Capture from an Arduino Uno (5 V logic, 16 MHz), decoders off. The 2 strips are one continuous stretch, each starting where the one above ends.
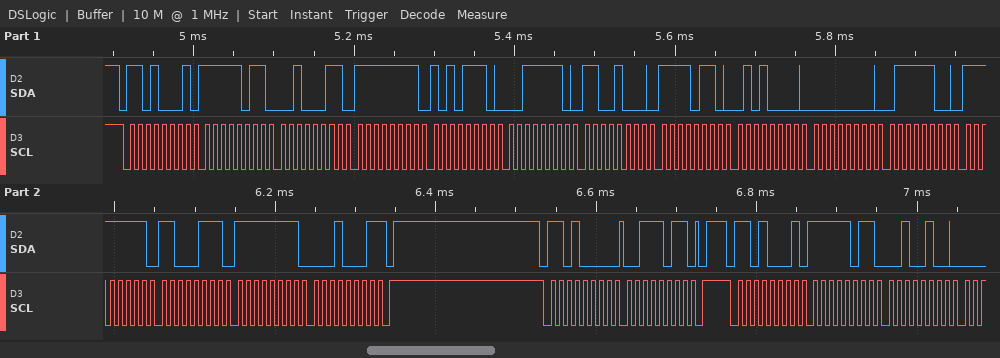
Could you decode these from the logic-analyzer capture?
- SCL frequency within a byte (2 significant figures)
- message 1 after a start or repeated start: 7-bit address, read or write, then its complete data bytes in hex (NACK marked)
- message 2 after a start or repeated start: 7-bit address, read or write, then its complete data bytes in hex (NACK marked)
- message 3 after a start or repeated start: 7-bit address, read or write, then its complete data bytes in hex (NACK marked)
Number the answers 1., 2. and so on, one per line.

1. 100 kHz
2. 0x68 read: FB 23 FF AE 3E C8 F6 50 00 7C FF C7 FF 11 NACK
3. 0x68 write: 3B
4. 0x68 read: FB 24
